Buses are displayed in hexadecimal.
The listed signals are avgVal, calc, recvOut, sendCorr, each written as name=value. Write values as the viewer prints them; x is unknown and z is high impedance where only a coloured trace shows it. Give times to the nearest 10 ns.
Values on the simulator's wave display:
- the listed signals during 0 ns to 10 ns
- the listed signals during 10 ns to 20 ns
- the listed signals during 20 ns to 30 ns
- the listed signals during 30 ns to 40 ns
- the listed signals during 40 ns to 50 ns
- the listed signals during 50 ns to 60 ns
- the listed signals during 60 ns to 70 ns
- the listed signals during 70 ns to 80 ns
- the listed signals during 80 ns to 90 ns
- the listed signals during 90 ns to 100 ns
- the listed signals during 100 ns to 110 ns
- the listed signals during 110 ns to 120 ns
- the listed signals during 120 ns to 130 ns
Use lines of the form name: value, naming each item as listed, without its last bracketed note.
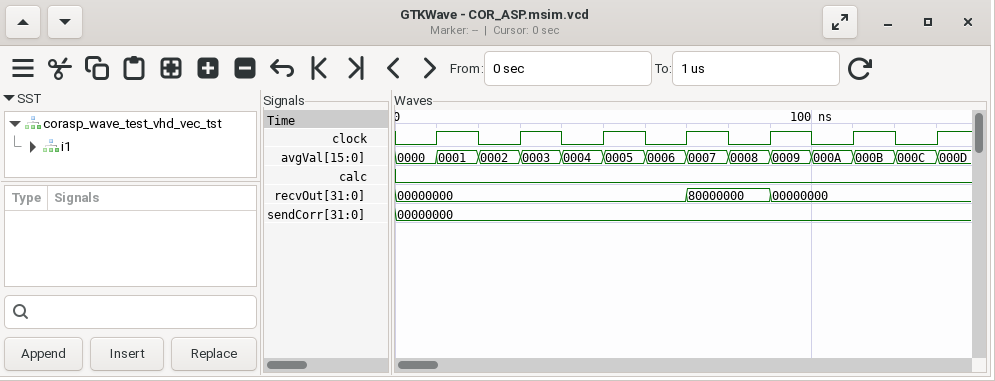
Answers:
the listed signals during 0 ns to 10 ns: avgVal=0000, calc=0, recvOut=00000000, sendCorr=00000000
the listed signals during 10 ns to 20 ns: avgVal=0001, calc=0, recvOut=00000000, sendCorr=00000000
the listed signals during 20 ns to 30 ns: avgVal=0002, calc=0, recvOut=00000000, sendCorr=00000000
the listed signals during 30 ns to 40 ns: avgVal=0003, calc=0, recvOut=00000000, sendCorr=00000000
the listed signals during 40 ns to 50 ns: avgVal=0004, calc=0, recvOut=00000000, sendCorr=00000000
the listed signals during 50 ns to 60 ns: avgVal=0005, calc=0, recvOut=00000000, sendCorr=00000000
the listed signals during 60 ns to 70 ns: avgVal=0006, calc=0, recvOut=00000000, sendCorr=00000000
the listed signals during 70 ns to 80 ns: avgVal=0007, calc=0, recvOut=80000000, sendCorr=00000000
the listed signals during 80 ns to 90 ns: avgVal=0008, calc=0, recvOut=80000000, sendCorr=00000000
the listed signals during 90 ns to 100 ns: avgVal=0009, calc=0, recvOut=00000000, sendCorr=00000000
the listed signals during 100 ns to 110 ns: avgVal=000A, calc=0, recvOut=00000000, sendCorr=00000000
the listed signals during 110 ns to 120 ns: avgVal=000B, calc=0, recvOut=00000000, sendCorr=00000000
the listed signals during 120 ns to 130 ns: avgVal=000C, calc=0, recvOut=00000000, sendCorr=00000000
